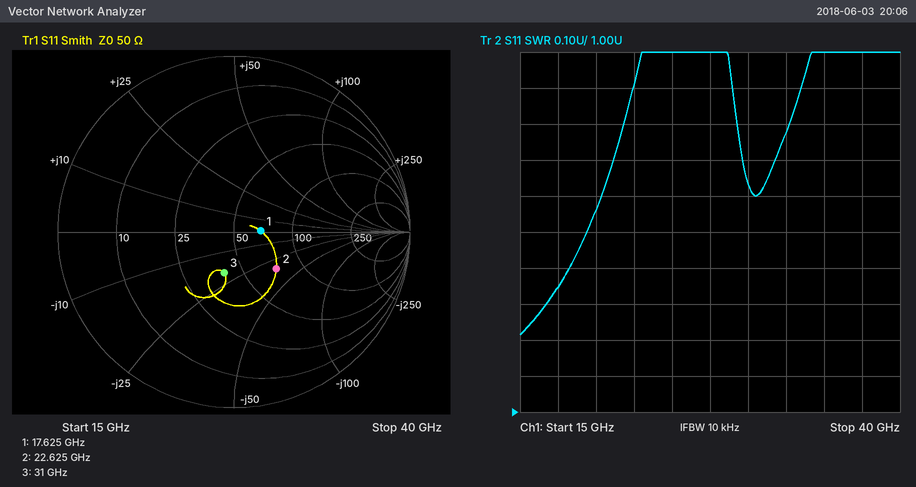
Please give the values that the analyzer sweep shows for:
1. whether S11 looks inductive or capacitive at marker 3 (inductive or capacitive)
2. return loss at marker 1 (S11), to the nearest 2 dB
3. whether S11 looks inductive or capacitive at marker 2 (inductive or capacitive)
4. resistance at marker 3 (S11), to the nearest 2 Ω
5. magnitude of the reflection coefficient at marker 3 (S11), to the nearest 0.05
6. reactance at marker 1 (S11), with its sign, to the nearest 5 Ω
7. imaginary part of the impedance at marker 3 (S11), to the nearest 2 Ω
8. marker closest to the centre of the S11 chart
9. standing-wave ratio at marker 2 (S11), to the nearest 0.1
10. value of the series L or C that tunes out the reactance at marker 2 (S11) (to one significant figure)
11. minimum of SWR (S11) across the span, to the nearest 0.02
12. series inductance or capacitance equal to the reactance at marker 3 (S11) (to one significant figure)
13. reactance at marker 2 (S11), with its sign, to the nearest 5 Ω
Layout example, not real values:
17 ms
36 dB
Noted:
capacitive
16 dB
capacitive
40 Ω
0.25
0 Ω
-20 Ω
marker 1
1.9
200 pH
1.22
300 fF
-35 Ω
